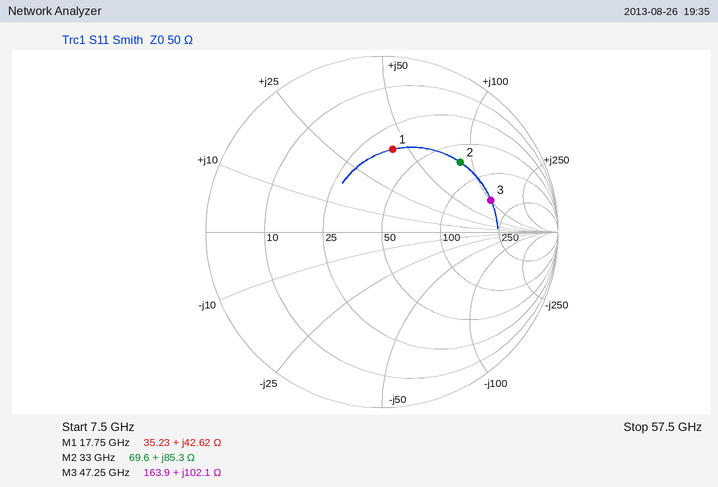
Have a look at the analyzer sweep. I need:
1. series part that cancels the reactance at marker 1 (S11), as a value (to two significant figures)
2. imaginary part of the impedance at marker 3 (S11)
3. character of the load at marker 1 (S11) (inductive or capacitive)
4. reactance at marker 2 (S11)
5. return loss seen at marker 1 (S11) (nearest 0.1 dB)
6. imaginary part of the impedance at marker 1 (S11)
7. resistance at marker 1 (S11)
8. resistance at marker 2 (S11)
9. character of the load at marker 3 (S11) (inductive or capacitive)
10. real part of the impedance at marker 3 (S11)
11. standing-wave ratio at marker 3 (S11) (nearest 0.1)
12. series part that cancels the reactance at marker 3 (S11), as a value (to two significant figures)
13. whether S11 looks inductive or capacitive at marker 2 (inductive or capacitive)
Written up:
210 fF
+102.1 Ω
inductive
+85.3 Ω
6.5 dB
+42.62 Ω
35.23 Ω
69.6 Ω
inductive
163.9 Ω
4.6
33 fF
inductive
